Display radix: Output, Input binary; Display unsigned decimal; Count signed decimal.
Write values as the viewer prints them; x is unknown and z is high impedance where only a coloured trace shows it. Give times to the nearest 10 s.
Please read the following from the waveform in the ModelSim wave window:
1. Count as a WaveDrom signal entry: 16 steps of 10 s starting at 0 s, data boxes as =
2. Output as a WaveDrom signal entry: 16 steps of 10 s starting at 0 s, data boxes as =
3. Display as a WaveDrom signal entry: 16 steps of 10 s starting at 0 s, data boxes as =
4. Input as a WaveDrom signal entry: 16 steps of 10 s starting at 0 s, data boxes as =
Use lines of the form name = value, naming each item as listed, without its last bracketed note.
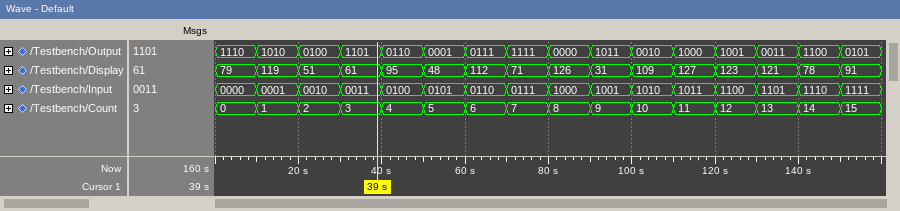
Count as a WaveDrom signal entry: 16 steps of 10 s starting at 0 s, data boxes as = = {name: 'Count', wave: '================', data: '0 1 2 3 4 5 6 7 8 9 10 11 12 13 14 15'}
Output as a WaveDrom signal entry: 16 steps of 10 s starting at 0 s, data boxes as = = {name: 'Output', wave: '================', data: '1110 1010 0100 1101 0110 0001 0111 1111 0000 1011 0010 1000 1001 0011 1100 0101'}
Display as a WaveDrom signal entry: 16 steps of 10 s starting at 0 s, data boxes as = = {name: 'Display', wave: '================', data: '79 119 51 61 95 48 112 71 126 31 109 127 123 121 78 91'}
Input as a WaveDrom signal entry: 16 steps of 10 s starting at 0 s, data boxes as = = {name: 'Input', wave: '================', data: '0000 0001 0010 0011 0100 0101 0110 0111 1000 1001 1010 1011 1100 1101 1110 1111'}
